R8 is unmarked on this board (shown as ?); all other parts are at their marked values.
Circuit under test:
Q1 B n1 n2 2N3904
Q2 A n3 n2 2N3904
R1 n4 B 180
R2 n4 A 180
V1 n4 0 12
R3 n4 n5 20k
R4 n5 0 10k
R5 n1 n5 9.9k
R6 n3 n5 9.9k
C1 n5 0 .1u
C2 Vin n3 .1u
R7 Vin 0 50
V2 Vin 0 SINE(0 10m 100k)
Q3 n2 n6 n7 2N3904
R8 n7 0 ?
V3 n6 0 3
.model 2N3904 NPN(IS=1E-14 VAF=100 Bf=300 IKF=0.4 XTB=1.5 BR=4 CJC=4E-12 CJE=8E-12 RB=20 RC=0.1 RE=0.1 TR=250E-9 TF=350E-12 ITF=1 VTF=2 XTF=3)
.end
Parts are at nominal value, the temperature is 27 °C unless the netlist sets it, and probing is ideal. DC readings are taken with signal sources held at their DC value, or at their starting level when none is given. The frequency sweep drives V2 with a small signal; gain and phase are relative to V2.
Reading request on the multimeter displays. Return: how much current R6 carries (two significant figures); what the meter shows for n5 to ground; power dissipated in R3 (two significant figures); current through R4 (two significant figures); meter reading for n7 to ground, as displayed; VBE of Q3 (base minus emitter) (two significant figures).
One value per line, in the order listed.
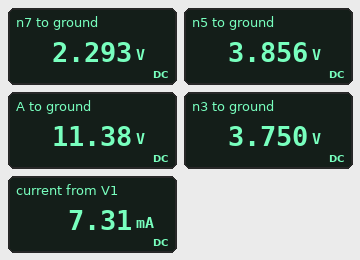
11 µA
3.856 V
3.3 mW
390 µA
2.293 V
710 mV
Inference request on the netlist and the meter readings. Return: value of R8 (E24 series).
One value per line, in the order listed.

330 Ω
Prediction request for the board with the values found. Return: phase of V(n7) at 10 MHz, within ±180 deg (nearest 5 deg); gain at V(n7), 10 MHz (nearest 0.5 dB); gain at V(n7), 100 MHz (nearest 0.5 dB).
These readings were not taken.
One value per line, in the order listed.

85 deg
-46.5 dB
-26.5 dB
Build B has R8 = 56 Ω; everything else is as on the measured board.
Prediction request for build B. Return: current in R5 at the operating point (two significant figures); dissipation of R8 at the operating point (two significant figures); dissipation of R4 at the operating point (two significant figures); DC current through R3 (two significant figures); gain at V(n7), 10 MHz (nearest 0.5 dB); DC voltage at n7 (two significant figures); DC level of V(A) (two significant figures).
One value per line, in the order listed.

49 µA
78 mW
1.1 mW
430 µA
-1.5 dB
2.1 V
9.3 V
